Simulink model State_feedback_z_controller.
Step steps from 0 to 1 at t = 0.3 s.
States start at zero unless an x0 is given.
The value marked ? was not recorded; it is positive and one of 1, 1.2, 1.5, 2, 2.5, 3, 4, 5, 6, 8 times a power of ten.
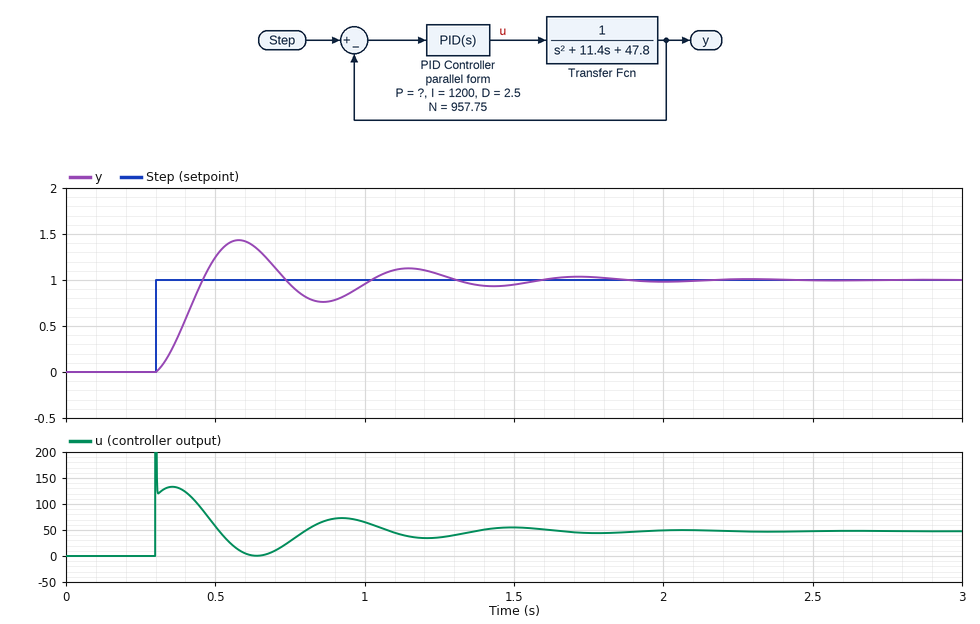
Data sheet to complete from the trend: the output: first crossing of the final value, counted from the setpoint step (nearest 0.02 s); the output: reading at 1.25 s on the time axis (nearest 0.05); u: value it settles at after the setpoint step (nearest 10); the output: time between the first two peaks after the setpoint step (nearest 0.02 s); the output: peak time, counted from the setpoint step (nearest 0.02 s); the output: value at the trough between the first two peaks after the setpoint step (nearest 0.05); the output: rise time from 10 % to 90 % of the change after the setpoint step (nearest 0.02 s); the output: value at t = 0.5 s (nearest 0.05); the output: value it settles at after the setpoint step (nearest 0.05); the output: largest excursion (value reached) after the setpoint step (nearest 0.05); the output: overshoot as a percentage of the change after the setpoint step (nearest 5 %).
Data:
0.16 s
1.05
50
0.56 s
0.28 s
0.75
0.12 s
1.25
1.00
1.45
45 %
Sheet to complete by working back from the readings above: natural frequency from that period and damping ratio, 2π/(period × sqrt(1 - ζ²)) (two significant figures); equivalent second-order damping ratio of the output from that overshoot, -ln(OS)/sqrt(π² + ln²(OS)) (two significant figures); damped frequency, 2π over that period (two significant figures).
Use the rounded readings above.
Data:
12 rad/s
0.25
11 rad/s
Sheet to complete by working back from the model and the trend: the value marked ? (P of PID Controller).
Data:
120
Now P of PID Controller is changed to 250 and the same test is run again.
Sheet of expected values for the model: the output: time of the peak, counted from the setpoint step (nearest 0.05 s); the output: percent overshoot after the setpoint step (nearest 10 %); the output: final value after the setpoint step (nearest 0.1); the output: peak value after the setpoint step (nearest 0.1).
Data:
0.20 s
30 %
1.0
1.3
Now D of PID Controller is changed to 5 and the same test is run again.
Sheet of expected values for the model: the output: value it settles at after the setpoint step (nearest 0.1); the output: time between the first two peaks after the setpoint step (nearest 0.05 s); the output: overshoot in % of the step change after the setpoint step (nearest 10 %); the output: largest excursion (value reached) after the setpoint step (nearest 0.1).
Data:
1.0
0.60 s
30 %
1.3
